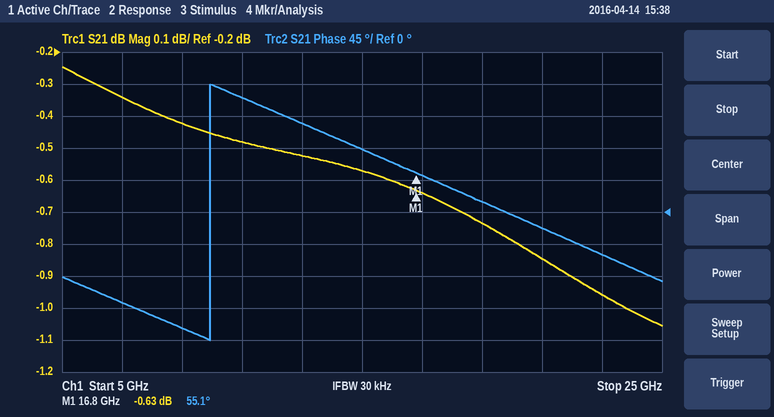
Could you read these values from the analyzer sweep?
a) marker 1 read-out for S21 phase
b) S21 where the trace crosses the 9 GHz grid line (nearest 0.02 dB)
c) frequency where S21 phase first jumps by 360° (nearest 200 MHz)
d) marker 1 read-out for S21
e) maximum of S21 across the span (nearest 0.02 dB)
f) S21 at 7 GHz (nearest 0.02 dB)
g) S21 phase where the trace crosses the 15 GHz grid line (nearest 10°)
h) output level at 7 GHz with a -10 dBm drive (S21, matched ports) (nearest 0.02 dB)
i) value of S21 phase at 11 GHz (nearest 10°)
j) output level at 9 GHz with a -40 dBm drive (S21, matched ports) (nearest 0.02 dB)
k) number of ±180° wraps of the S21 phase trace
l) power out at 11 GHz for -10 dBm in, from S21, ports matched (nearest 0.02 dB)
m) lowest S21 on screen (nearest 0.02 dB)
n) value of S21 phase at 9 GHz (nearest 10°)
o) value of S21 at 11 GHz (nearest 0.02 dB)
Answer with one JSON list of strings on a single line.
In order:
["55.1°", "-0.42 dB", "10.0 GHz", "-0.63 dB", "-0.24 dB", "-0.34 dB", "90°", "-10.34 dBm", "160°", "-40.42 dBm", "1", "-10.48 dBm", "-1.06 dB", "-160°", "-0.48 dB"]
